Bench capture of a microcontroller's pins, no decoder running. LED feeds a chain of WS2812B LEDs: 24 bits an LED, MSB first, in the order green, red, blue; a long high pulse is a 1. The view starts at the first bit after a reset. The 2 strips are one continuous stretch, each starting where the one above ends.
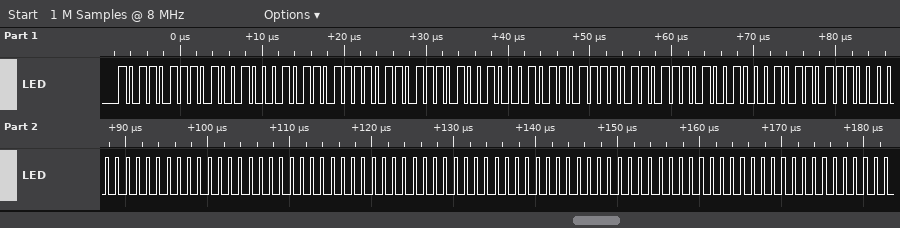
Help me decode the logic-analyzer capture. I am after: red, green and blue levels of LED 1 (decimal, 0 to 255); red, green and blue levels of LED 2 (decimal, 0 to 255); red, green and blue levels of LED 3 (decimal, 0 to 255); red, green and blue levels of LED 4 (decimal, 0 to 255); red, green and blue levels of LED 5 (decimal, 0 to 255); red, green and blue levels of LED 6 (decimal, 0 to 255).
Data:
72, 183, 183
72, 183, 183
72, 183, 183
0, 0, 0
0, 0, 0
0, 0, 0
